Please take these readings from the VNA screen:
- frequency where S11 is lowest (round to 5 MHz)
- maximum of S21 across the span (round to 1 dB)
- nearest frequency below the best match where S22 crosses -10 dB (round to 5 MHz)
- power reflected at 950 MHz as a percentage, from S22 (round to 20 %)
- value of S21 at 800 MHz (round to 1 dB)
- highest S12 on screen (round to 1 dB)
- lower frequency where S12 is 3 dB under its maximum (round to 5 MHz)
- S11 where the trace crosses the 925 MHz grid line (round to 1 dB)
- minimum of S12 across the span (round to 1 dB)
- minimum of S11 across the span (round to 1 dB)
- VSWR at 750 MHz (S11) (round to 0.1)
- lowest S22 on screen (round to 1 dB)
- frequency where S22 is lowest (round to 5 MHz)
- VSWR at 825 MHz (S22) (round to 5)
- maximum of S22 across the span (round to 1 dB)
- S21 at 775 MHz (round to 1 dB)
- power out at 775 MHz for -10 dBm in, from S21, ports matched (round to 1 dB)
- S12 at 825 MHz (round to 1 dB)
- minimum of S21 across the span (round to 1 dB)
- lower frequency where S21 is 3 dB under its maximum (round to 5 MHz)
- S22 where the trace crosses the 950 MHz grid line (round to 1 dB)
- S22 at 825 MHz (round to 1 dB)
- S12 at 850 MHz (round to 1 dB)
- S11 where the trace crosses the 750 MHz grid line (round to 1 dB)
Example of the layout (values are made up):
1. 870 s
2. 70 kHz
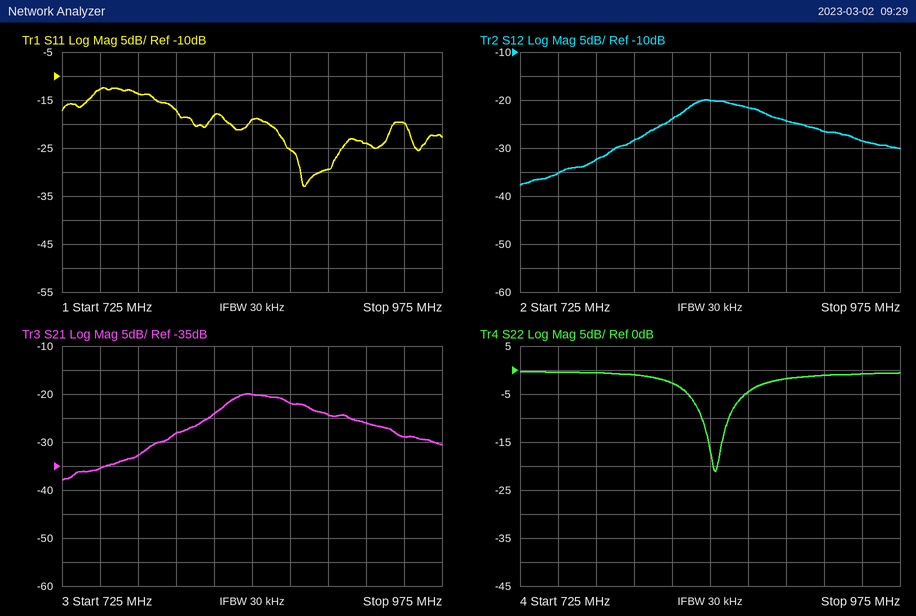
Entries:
1. 885 MHz
2. -20 dB
3. 845 MHz
4. 80 %
5. -28 dB
6. -20 dB
7. 830 MHz
8. -24 dB
9. -38 dB
10. -33 dB
11. 1.6
12. -21 dB
13. 855 MHz
14. 5
15. 0 dB
16. -33 dB
17. -43 dBm
18. -24 dB
19. -38 dB
20. 830 MHz
21. -1 dB
22. -3 dB
23. -20 dB
24. -13 dB
